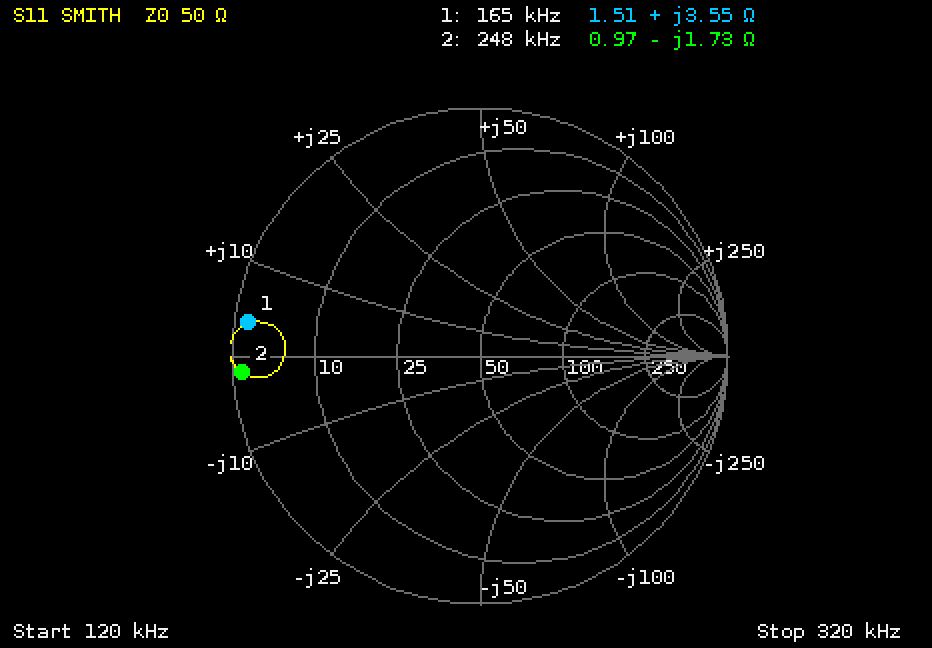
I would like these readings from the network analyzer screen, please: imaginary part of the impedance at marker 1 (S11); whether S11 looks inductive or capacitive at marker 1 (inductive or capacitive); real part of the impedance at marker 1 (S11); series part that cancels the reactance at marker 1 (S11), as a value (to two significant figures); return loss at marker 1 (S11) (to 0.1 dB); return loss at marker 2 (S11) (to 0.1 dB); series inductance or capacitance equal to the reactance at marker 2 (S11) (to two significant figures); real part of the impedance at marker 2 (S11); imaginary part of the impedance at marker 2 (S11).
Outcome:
+3.55 Ω
inductive
1.51 Ω
270 nF
0.5 dB
0.3 dB
370 nF
0.97 Ω
-1.73 Ω
